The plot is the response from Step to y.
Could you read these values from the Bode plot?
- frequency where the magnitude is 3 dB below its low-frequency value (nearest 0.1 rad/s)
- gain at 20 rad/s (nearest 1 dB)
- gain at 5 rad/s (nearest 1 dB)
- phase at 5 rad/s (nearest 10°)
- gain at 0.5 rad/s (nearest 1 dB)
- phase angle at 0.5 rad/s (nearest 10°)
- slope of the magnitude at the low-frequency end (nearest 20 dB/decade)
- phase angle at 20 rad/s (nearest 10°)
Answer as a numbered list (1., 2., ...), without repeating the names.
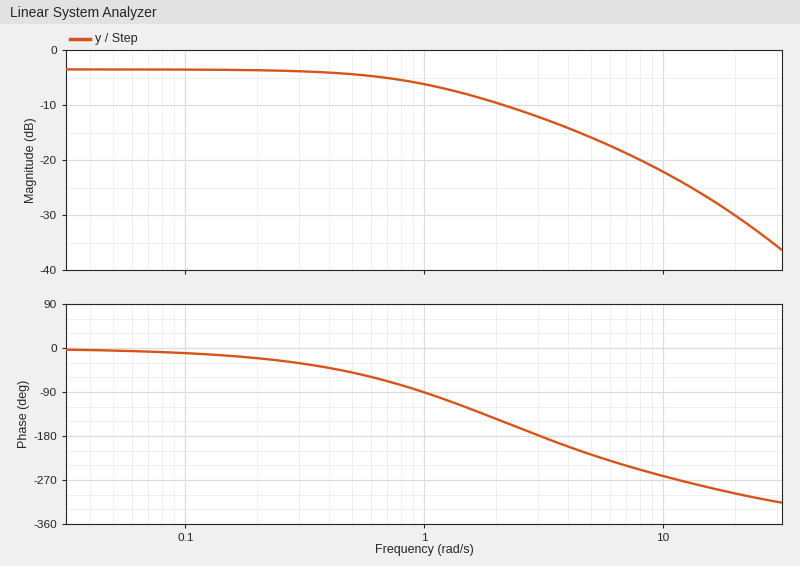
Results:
1. 1.1 rad/s
2. -30 dB
3. -16 dB
4. -220°
5. -4 dB
6. -50°
7. 0 dB/decade
8. -300°
